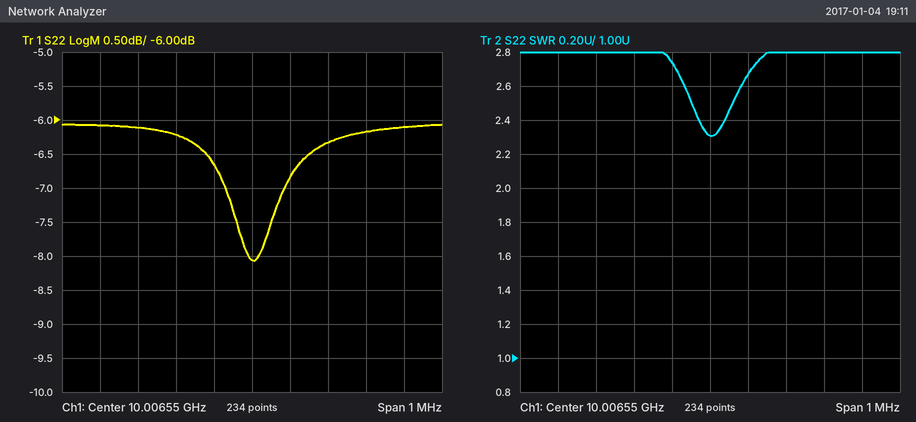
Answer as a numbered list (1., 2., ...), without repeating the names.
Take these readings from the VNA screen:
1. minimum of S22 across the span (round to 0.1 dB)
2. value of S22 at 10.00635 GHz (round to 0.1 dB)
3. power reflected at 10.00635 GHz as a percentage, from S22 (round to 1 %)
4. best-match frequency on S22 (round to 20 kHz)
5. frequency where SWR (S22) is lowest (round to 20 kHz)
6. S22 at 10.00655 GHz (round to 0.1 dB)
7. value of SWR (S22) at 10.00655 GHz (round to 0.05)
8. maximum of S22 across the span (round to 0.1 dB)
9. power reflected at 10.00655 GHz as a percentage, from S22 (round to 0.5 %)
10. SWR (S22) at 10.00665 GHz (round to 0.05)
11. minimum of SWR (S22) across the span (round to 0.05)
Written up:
1. -8.1 dB
2. -6.2 dB
3. 24 %
4. 10.00656 GHz
5. 10.00656 GHz
6. -8.1 dB
7. 2.30
8. -6.1 dB
9. 15.5 %
10. 2.65
11. 2.30
